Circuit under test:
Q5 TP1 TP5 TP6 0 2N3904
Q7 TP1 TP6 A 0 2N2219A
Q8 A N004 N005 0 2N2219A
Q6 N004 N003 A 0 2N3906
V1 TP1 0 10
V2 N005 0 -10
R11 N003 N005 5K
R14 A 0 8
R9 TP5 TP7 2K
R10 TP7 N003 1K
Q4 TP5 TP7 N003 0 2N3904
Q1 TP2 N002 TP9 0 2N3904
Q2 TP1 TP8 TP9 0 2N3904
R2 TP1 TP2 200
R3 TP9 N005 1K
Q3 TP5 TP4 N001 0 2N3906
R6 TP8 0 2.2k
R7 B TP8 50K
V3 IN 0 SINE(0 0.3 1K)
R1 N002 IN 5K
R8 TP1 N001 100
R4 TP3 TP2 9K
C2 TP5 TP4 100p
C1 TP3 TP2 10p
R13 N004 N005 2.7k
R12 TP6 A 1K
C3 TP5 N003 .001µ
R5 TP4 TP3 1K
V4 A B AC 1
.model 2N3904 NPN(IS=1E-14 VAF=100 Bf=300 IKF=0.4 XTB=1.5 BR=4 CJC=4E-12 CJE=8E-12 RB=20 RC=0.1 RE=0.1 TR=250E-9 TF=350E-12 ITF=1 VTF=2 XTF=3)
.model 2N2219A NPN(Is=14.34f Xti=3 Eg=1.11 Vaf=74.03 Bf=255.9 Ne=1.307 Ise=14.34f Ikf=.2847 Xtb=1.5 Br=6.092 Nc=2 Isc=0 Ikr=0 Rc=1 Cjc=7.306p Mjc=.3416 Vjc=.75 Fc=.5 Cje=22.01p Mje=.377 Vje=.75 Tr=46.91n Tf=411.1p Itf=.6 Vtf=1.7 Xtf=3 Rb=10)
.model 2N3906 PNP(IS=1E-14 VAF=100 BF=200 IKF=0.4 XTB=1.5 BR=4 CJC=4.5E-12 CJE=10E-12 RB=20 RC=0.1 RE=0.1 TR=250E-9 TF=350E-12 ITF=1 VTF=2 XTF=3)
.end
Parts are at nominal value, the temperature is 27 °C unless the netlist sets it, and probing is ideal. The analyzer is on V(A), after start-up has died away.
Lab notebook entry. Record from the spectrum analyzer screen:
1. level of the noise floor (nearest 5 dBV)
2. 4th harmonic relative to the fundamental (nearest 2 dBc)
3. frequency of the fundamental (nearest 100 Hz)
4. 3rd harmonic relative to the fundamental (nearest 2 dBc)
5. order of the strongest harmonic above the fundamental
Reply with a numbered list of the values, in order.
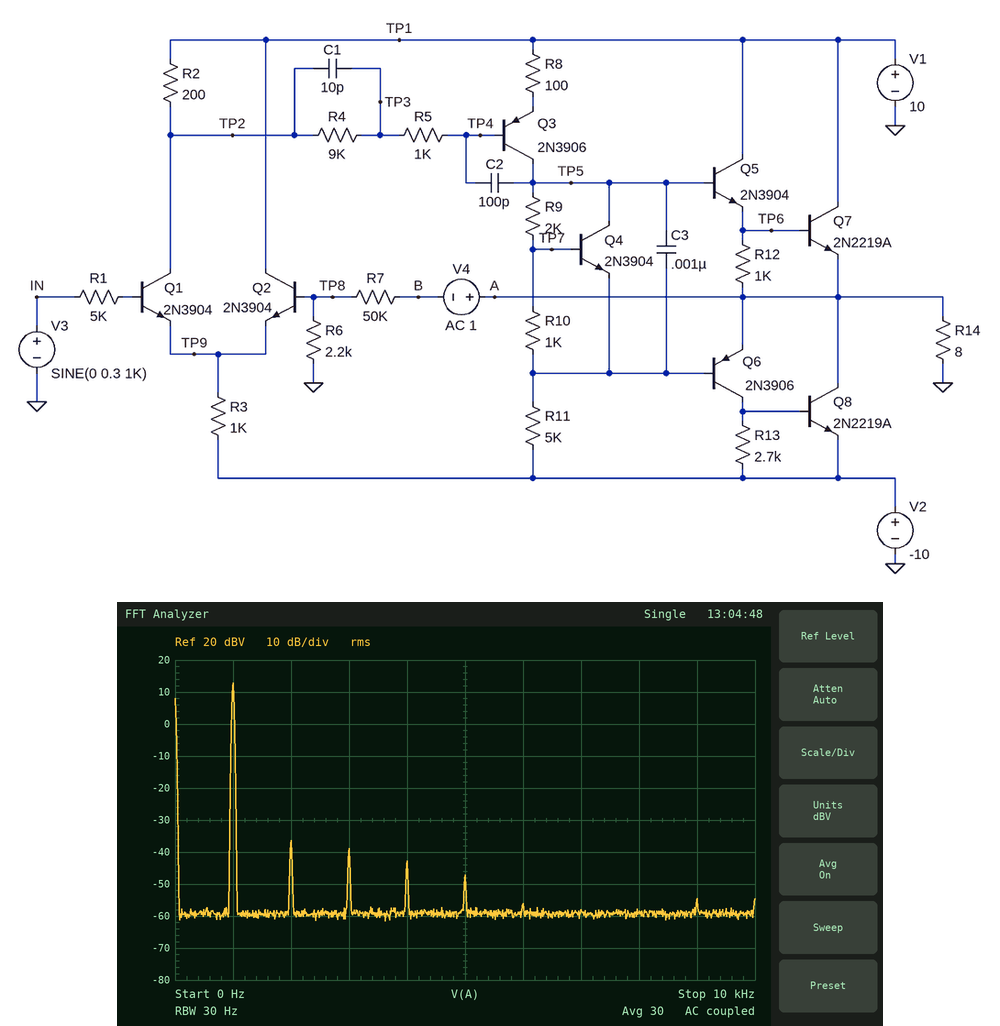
1. -60 dBV
2. -56 dBc
3. 1.0 kHz
4. -52 dBc
5. 2
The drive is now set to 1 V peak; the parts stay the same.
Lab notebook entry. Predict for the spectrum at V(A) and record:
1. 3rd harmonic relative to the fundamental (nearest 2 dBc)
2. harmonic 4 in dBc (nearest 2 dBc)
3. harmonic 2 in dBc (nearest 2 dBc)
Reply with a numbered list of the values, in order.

1. -12 dBc
2. -36 dBc
3. -32 dBc
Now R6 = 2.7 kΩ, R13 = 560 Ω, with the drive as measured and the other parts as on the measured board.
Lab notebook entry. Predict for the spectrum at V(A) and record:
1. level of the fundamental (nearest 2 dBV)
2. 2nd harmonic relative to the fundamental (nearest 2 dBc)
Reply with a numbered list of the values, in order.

1. 12 dBV
2. -58 dBc
